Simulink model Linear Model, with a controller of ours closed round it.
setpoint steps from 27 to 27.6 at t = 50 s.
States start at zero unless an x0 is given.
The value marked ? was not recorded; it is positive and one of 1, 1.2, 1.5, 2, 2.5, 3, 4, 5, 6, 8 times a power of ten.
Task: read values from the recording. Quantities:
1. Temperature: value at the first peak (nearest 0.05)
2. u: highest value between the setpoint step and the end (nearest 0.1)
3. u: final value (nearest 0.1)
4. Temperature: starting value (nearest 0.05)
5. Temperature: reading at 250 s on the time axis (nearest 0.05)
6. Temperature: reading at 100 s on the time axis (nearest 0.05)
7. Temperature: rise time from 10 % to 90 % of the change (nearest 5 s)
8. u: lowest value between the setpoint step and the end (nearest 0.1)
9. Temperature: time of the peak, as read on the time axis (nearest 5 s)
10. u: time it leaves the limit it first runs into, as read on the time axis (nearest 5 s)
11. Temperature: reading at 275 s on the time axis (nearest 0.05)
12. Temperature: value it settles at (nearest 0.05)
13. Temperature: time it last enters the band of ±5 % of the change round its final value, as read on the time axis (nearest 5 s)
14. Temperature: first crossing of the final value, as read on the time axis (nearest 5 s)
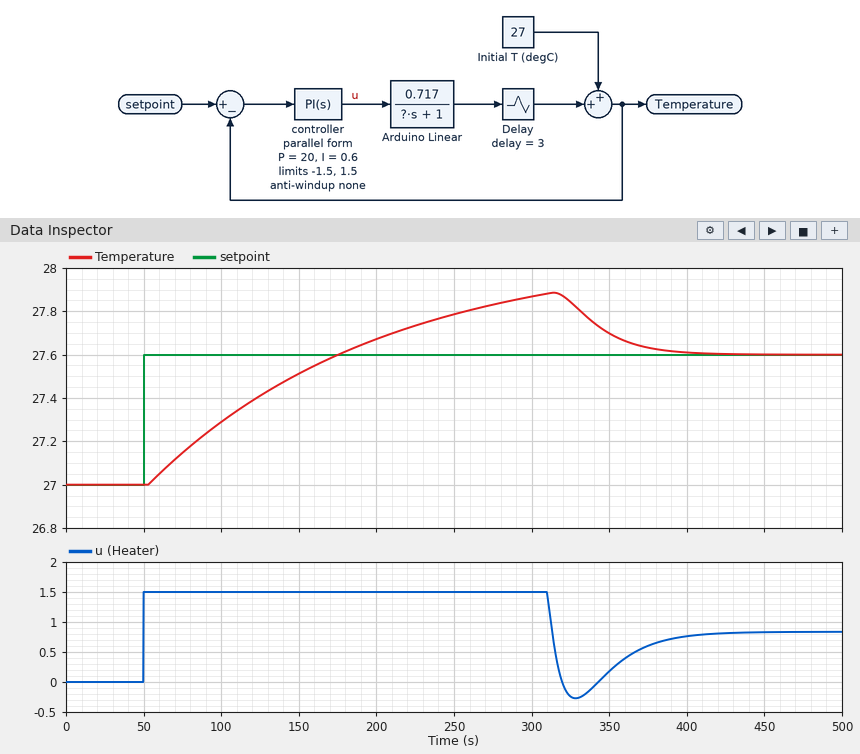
27.90
1.5
0.8
27.00
27.80
27.30
95 s
-0.3
315 s
310 s
27.85
27.60
375 s
175 s
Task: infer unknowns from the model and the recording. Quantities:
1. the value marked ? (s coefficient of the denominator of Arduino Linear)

150
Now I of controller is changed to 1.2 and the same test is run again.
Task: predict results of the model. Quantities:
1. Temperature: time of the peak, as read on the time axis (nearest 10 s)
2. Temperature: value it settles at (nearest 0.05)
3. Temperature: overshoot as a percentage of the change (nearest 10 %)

330 s
27.60
50 %
